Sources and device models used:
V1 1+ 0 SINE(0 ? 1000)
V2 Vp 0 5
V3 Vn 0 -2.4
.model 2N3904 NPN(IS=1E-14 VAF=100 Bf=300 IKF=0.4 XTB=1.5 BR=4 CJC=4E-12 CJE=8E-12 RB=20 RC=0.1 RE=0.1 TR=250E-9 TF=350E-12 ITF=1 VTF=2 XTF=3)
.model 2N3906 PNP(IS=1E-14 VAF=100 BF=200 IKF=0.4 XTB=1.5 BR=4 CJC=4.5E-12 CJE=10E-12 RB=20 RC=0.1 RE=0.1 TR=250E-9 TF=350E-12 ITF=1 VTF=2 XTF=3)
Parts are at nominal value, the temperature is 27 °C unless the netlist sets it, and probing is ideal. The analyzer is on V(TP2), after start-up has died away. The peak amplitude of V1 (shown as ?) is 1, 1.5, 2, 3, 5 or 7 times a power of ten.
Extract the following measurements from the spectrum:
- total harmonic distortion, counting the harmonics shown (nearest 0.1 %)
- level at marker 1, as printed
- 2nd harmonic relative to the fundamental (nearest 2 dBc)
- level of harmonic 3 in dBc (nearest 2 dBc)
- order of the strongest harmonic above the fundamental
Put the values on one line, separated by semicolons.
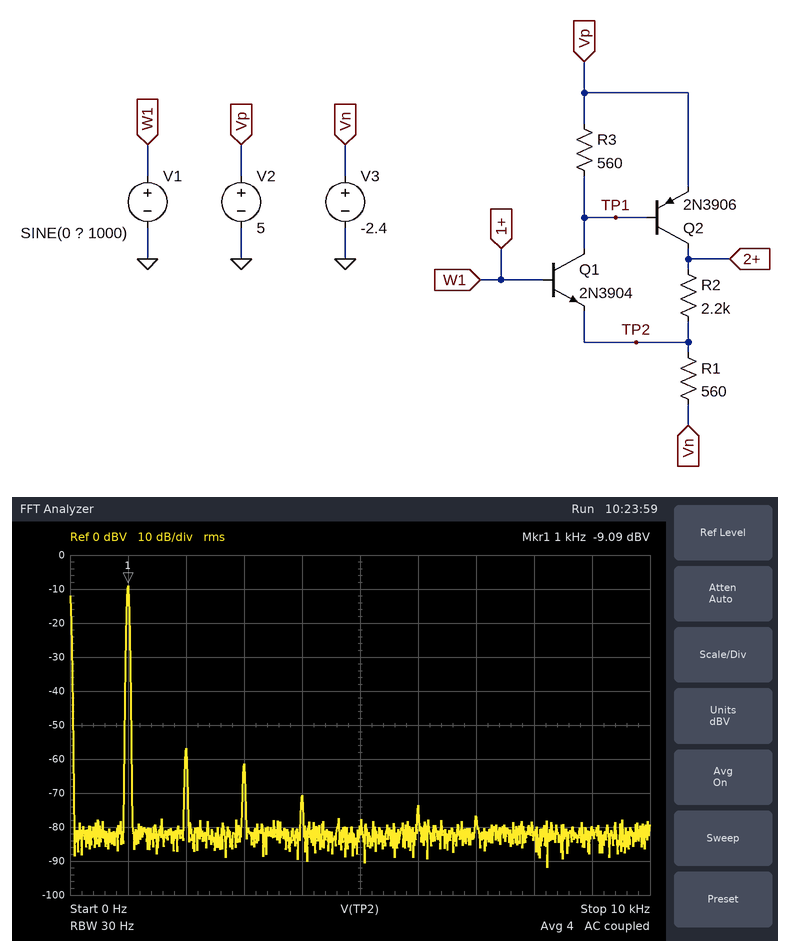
0.5 %; -9.09 dBV; -48 dBc; -52 dBc; 2
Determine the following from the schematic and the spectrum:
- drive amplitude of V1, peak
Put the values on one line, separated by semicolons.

500 mV
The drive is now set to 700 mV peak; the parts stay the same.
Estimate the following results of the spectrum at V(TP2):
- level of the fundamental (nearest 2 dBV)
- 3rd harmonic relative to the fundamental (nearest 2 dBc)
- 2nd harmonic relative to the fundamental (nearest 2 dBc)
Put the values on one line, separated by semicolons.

-6 dBV; -54 dBc; -46 dBc
